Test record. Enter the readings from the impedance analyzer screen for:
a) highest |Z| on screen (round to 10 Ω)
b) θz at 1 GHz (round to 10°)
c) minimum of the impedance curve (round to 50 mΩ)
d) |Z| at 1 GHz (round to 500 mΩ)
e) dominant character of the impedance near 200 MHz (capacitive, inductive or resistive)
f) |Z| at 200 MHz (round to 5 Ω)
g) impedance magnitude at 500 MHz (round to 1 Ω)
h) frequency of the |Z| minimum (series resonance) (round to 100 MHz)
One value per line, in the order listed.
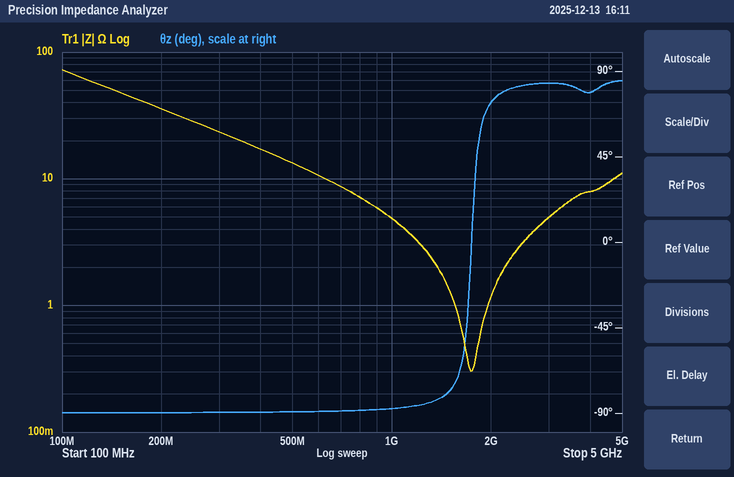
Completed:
70 Ω
-90°
300 mΩ
5.0 Ω
capacitive
35 Ω
13 Ω
1.7 GHz
